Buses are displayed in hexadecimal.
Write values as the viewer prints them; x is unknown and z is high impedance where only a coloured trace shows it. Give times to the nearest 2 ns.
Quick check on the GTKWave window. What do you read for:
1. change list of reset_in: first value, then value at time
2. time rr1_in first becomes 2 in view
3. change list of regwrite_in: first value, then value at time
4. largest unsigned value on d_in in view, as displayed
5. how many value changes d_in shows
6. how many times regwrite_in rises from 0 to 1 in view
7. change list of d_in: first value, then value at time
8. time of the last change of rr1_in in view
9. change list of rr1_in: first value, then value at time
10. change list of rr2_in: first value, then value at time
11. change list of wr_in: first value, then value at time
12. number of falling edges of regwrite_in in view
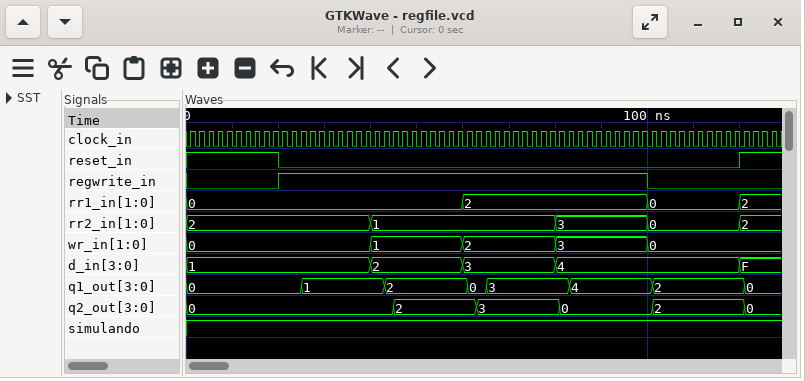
1, 0 at 20 ns, 1 at 120 ns
60 ns
0, 1 at 20 ns, 0 at 100 ns
F
4
1
1, 2 at 40 ns, 3 at 60 ns, 4 at 80 ns, F at 120 ns
120 ns
0, 2 at 60 ns, 0 at 100 ns, 2 at 120 ns
2, 1 at 40 ns, 3 at 80 ns, 0 at 100 ns, 2 at 120 ns
0, 1 at 40 ns, 2 at 60 ns, 3 at 80 ns, 0 at 100 ns
1
